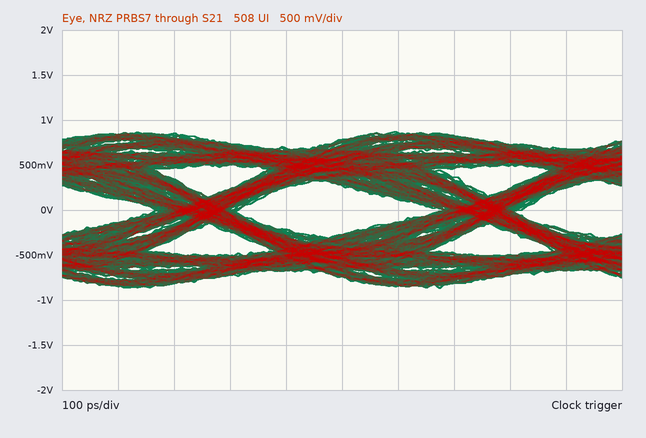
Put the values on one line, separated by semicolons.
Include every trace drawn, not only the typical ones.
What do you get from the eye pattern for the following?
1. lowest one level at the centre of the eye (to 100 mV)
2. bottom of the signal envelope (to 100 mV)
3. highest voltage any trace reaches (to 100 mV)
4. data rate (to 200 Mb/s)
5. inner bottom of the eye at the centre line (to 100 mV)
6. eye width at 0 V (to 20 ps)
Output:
300 mV; -900 mV; 900 mV; 2.0 Gb/s; -300 mV; 360 ps
